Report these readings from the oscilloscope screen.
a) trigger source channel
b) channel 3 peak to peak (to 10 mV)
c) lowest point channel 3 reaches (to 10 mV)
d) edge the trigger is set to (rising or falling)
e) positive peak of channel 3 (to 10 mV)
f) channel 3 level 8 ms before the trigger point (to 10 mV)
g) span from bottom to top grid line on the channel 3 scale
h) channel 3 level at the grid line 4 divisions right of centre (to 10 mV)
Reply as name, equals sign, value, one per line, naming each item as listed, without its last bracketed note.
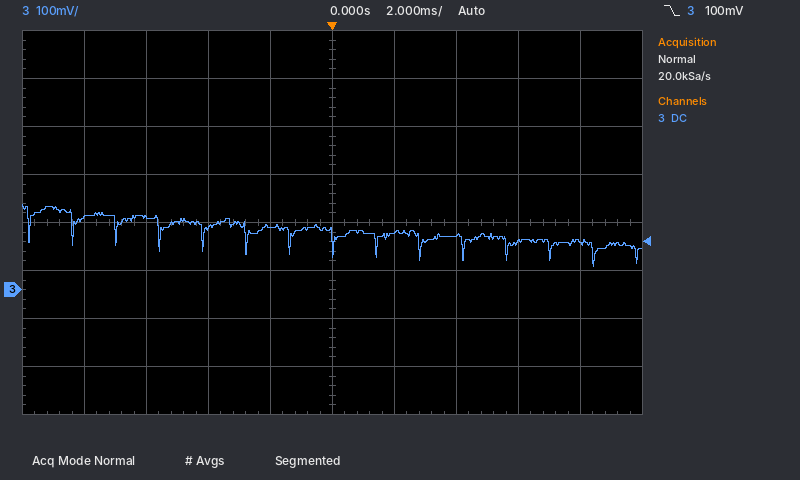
trigger source channel = channel 3
channel 3 peak to peak = 130 mV
lowest point channel 3 reaches = 50 mV
edge the trigger is set to = falling
positive peak of channel 3 = 180 mV
channel 3 level 8 ms before the trigger point = 150 mV
span from bottom to top grid line on the channel 3 scale = 800 mV
channel 3 level at the grid line 4 divisions right of centre = 100 mV
